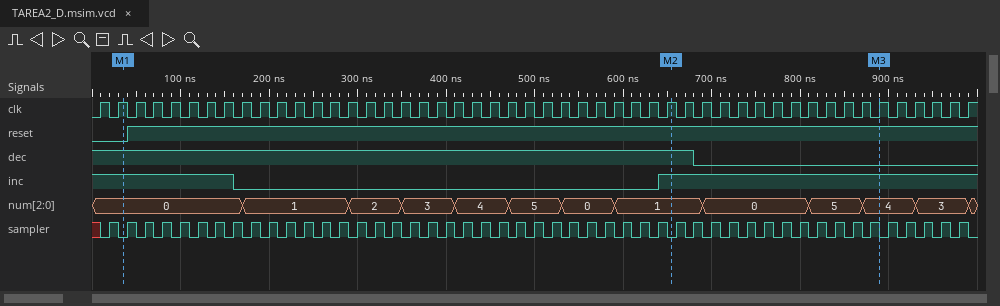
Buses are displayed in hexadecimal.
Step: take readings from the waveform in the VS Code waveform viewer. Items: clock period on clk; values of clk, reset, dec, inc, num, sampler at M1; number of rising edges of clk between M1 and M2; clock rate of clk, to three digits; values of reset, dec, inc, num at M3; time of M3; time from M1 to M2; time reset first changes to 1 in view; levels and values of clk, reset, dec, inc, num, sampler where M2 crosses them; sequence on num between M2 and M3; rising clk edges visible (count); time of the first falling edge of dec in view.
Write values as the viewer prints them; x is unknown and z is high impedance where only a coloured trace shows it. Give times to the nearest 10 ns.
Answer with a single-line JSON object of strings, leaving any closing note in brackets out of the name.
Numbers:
{"clock period on clk": "20 ns", "values of clk, reset, dec, inc, num, sampler at M1": "clk=1, reset=0, dec=1, inc=1, num=0, sampler=0", "number of rising edges of clk between M1 and M2": "31", "clock rate of clk, to three digits": "50.0 MHz", "values of reset, dec, inc, num at M3": "reset=1, dec=0, inc=1, num=4", "time of M3": "890 ns", "time from M1 to M2": "620 ns", "time reset first changes to 1 in view": "40 ns", "levels and values of clk, reset, dec, inc, num, sampler where M2 crosses them": "clk=1, reset=1, dec=1, inc=1, num=1, sampler=0", "sequence on num between M2 and M3": "1, 0, 5, 4", "rising clk edges visible": "50", "time of the first falling edge of dec in view": "680 ns"}
